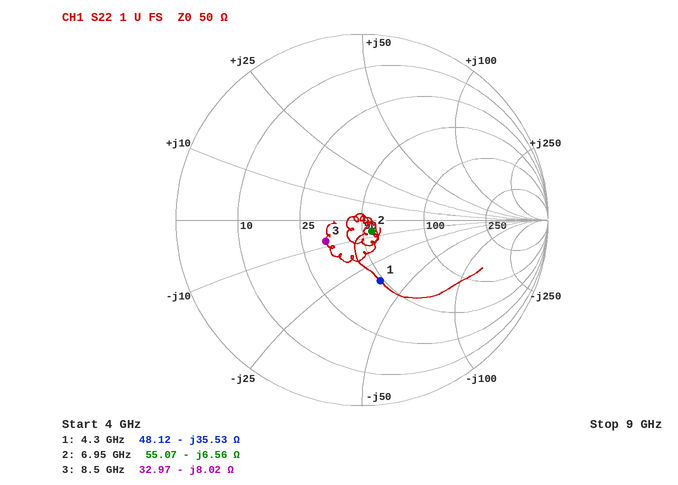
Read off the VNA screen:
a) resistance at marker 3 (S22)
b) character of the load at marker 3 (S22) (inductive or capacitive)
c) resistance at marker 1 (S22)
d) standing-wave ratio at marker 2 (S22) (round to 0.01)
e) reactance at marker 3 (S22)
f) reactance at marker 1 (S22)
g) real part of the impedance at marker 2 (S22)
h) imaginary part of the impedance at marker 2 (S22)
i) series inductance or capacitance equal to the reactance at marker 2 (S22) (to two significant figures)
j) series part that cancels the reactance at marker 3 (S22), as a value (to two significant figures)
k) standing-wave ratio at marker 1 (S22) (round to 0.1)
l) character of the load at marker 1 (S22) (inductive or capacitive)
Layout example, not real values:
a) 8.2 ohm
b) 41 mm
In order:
a) 32.97 Ω
b) capacitive
c) 48.12 Ω
d) 1.17
e) -8.02 Ω
f) -35.53 Ω
g) 55.07 Ω
h) -6.56 Ω
i) 3.5 pF
j) 150 pH
k) 2.0
l) capacitive
